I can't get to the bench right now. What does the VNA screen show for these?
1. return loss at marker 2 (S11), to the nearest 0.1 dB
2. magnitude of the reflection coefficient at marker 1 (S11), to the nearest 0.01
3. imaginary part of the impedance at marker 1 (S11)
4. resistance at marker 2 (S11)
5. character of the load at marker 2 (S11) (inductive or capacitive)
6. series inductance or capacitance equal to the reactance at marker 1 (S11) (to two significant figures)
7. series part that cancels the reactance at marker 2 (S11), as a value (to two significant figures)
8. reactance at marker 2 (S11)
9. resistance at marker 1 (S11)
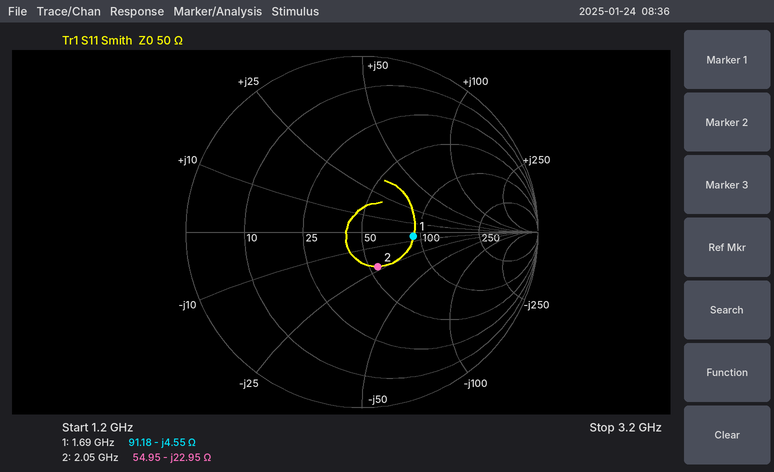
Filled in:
13.2 dB
0.29
-4.55 Ω
54.95 Ω
capacitive
21 pF
1.8 nH
-22.95 Ω
91.18 Ω
